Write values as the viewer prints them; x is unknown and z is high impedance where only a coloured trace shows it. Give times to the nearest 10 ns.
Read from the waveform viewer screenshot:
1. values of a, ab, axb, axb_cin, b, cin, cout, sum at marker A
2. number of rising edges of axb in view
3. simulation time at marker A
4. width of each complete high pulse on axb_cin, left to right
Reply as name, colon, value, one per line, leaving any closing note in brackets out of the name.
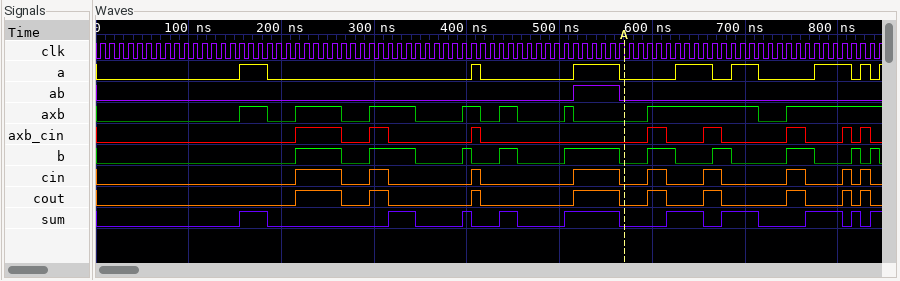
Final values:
values of a, ab, axb, axb_cin, b, cin, cout, sum at marker A: a=0, ab=0, axb=0, axb_cin=0, b=0, cin=0, cout=0, sum=0
number of rising edges of axb in view: 8
simulation time at marker A: 570 ns
width of each complete high pulse on axb_cin, left to right: 50 ns, 20 ns, 10 ns, 20 ns, 20 ns, 20 ns, 10 ns, 10 ns
